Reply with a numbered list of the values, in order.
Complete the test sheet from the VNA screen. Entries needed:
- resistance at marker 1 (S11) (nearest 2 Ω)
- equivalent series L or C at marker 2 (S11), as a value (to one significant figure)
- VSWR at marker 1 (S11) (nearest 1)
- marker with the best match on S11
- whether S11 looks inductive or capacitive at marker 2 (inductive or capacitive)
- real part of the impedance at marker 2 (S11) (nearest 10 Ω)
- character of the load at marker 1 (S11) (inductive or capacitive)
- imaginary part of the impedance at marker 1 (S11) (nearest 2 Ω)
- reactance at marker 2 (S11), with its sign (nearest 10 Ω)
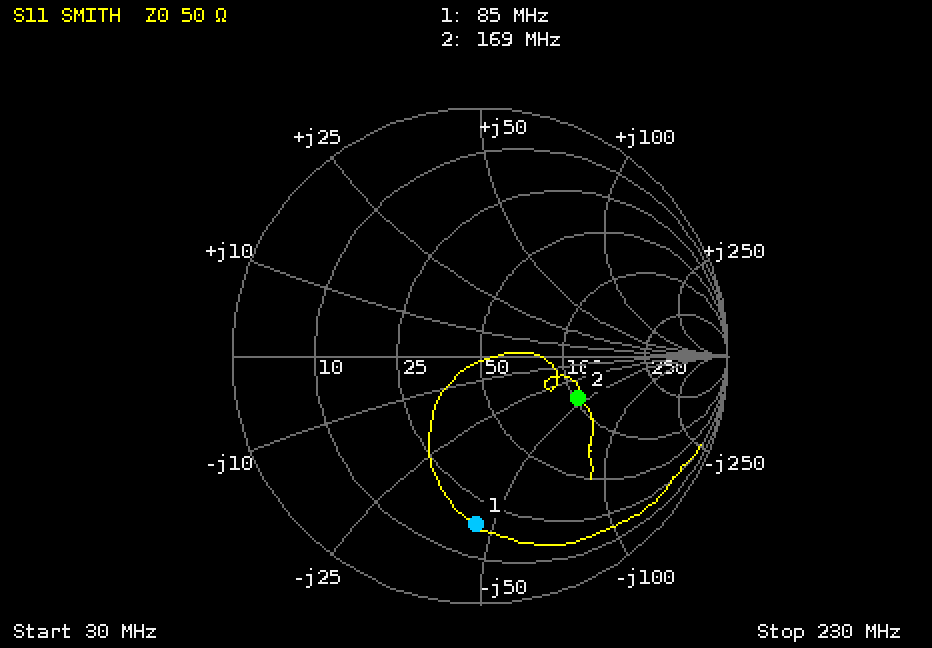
1. 18 Ω
2. 20 pF
3. 5
4. marker 2
5. capacitive
6. 100 Ω
7. capacitive
8. -46 Ω
9. -40 Ω
